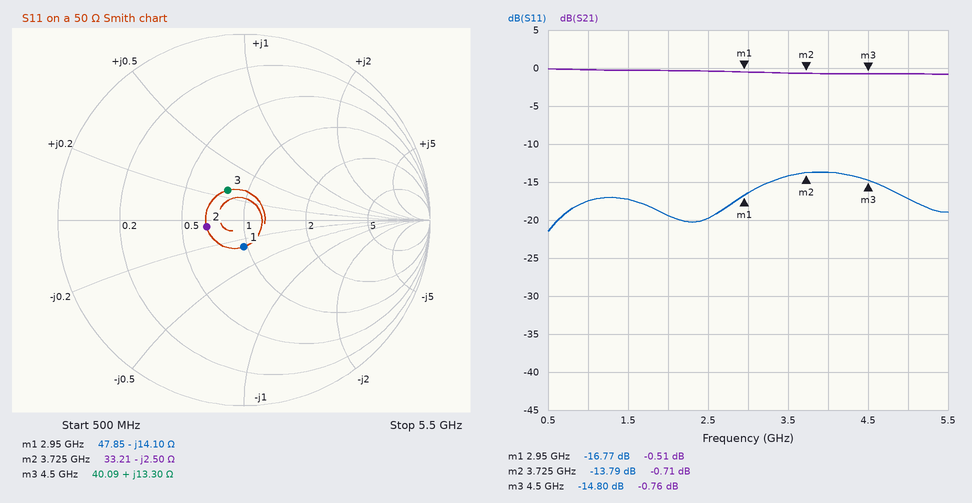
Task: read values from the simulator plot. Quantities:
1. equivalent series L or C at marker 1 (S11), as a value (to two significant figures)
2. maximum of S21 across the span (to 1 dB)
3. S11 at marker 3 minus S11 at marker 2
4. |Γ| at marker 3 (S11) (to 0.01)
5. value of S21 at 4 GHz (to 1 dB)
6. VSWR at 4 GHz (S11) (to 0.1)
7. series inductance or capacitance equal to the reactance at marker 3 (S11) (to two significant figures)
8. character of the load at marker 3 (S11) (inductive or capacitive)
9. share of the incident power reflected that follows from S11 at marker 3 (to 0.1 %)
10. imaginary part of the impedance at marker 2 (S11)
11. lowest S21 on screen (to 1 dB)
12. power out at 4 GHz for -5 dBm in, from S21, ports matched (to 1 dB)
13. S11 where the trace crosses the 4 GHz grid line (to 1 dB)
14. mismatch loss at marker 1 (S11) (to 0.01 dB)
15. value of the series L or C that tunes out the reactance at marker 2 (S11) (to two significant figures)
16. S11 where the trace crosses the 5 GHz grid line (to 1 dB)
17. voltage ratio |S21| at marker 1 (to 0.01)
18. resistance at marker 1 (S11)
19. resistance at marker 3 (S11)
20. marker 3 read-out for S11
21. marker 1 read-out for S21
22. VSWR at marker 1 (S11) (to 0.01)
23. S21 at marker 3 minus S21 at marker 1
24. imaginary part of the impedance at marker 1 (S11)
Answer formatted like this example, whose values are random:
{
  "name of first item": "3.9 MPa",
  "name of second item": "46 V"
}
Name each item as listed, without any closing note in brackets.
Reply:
{
  "equivalent series L or C at marker 1 (S11), as a value": "3.8 pF",
  "maximum of S21 across the span": "0 dB",
  "S11 at marker 3 minus S11 at marker 2": "-1.01 dB",
  "|Γ| at marker 3 (S11)": "0.18",
  "value of S21 at 4 GHz": "-1 dB",
  "VSWR at 4 GHz (S11)": "1.5",
  "series inductance or capacitance equal to the reactance at marker 3 (S11)": "470 pH",
  "character of the load at marker 3 (S11)": "inductive",
  "share of the incident power reflected that follows from S11 at marker 3": "3.3 %",
  "imaginary part of the impedance at marker 2": "-2.50 Ω",
  "lowest S21 on screen": "-1 dB",
  "power out at 4 GHz for -5 dBm in, from S21, ports matched": "-6 dBm",
  "S11 where the trace crosses the 4 GHz grid line": "-14 dB",
  "mismatch loss at marker 1 (S11)": "0.09 dB",
  "value of the series L or C that tunes out the reactance at marker 2 (S11)": "110 pH",
  "S11 where the trace crosses the 5 GHz grid line": "-17 dB",
  "voltage ratio |S21| at marker 1": "0.94",
  "resistance at marker 1": "47.85 Ω",
  "resistance at marker 3": "40.09 Ω",
  "marker 3 read-out for S11": "-14.80 dB",
  "marker 1 read-out for S21": "-0.51 dB",
  "VSWR at marker 1 (S11)": "1.34",
  "S21 at marker 3 minus S21 at marker 1": "-0.25 dB",
  "imaginary part of the impedance at marker 1": "-14.10 Ω"
}
